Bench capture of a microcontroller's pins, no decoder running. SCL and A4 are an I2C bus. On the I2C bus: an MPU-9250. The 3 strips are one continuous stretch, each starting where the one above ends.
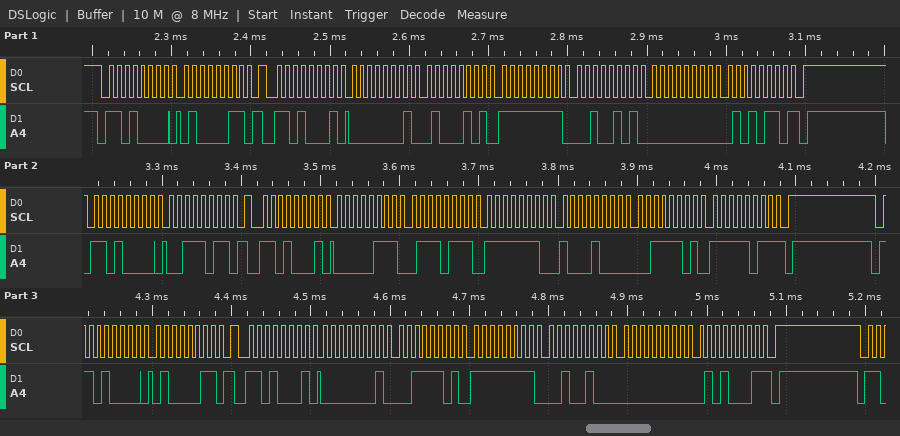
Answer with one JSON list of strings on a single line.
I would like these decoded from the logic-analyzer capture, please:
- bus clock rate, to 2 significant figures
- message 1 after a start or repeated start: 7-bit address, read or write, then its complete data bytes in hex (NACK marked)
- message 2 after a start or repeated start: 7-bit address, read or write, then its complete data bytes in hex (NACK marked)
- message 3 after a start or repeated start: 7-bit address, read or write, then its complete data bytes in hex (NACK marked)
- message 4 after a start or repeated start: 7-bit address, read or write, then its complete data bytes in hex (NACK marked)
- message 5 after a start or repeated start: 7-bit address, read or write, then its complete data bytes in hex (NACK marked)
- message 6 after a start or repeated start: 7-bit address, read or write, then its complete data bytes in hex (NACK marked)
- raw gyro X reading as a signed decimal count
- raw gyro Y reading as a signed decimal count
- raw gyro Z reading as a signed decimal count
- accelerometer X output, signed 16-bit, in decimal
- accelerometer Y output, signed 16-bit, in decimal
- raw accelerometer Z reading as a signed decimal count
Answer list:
["100 kHz", "0x68 write: 43", "0x68 read: 01 45 FF 25 00 56 NACK", "0x68 write: 3B", "0x68 read: 07 77 FE 88 3D FB NACK", "0x68 write: 43", "0x68 read: 01 3D FF 24 00 51 NACK", "325", "-219", "86", "1911", "-376", "15867"]
